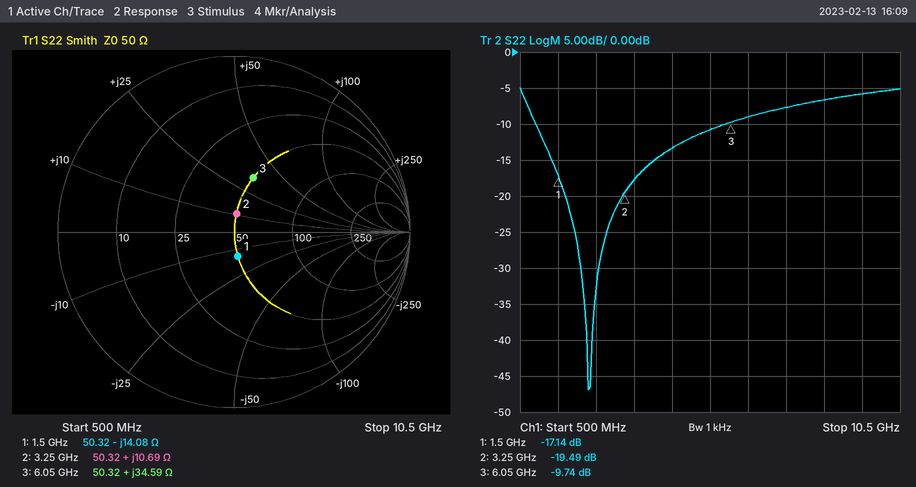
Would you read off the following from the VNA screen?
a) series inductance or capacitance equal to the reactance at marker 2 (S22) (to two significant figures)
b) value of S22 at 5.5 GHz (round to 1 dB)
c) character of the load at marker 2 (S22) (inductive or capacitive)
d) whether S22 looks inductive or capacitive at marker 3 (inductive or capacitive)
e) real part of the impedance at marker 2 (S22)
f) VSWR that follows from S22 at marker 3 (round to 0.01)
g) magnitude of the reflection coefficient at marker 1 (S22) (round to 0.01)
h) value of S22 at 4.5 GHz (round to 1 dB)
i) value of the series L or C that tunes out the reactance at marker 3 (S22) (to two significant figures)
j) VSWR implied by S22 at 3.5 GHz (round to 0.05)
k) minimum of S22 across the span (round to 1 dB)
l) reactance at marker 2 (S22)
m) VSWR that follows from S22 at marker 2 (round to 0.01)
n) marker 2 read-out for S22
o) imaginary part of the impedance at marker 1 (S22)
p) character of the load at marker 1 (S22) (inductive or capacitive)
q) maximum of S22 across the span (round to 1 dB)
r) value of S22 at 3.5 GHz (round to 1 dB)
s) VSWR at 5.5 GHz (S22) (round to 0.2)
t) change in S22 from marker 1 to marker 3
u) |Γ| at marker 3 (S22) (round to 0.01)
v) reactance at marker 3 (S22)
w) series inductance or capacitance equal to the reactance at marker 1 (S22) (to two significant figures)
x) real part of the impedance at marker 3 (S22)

520 pH
-11 dB
inductive
inductive
50.32 Ω
1.97
0.14
-13 dB
760 fF
1.30
-47 dB
+10.69 Ω
1.24
-19.49 dB
-14.08 Ω
capacitive
-5 dB
-18 dB
1.8
7.40 dB
0.33
+34.59 Ω
7.5 pF
50.32 Ω
